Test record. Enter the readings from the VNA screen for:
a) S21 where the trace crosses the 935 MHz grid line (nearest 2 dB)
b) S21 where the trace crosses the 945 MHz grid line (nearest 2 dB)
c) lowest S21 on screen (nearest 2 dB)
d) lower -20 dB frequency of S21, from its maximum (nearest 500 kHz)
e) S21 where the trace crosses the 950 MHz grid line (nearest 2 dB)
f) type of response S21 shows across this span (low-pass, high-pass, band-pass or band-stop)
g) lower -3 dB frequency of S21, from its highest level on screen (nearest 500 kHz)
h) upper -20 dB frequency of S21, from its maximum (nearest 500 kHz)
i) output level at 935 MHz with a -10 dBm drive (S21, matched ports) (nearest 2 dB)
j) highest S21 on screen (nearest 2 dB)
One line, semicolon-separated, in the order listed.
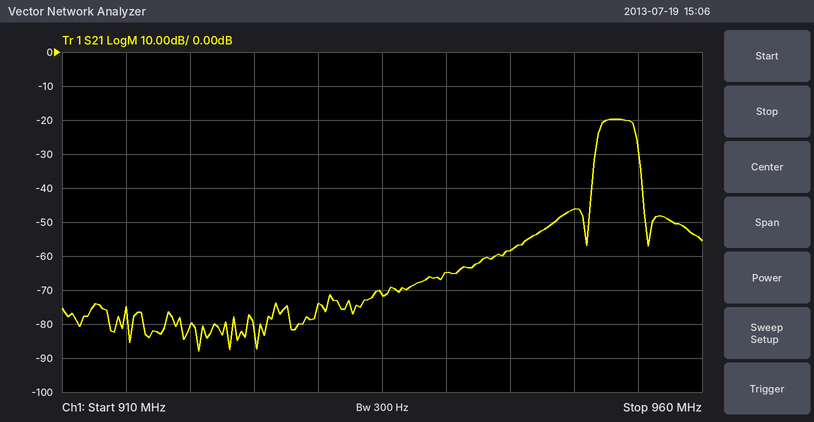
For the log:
-72 dB; -58 dB; -88 dB; 951.5 MHz; -46 dB; band-pass; 952.0 MHz; 955.5 MHz; -82 dBm; -20 dB
